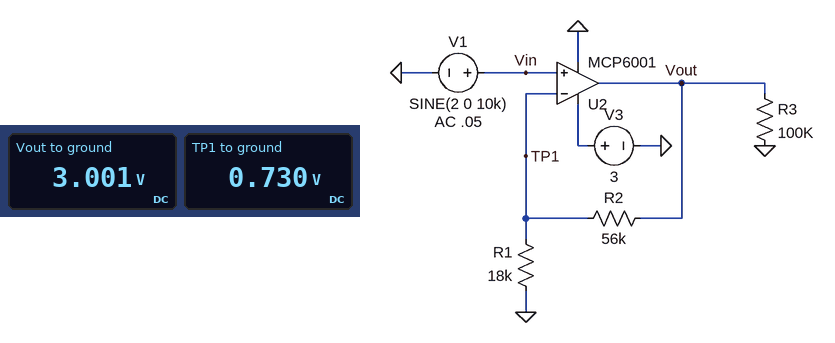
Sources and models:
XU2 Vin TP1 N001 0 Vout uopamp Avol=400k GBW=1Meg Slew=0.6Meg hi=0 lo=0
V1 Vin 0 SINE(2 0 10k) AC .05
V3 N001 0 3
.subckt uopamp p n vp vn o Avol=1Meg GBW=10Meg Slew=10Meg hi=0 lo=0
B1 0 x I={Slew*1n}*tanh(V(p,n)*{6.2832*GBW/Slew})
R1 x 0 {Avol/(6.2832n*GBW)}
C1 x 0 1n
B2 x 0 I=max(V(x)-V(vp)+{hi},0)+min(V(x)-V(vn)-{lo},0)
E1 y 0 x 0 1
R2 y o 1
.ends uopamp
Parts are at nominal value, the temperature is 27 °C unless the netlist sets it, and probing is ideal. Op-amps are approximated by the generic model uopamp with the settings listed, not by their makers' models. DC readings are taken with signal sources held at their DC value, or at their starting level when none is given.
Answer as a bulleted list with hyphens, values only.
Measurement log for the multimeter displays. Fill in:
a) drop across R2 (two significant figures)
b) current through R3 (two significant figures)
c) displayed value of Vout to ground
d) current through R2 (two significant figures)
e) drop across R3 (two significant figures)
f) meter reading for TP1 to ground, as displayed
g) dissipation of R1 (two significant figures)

- 2.3 V
- 30 µA
- 3.001 V
- 41 µA
- 3.0 V
- 0.730 V
- 30 µW
